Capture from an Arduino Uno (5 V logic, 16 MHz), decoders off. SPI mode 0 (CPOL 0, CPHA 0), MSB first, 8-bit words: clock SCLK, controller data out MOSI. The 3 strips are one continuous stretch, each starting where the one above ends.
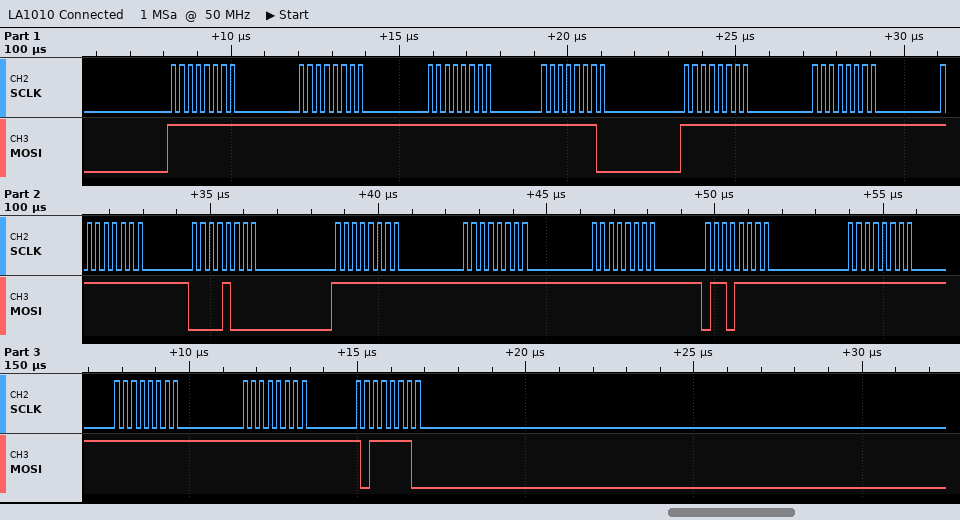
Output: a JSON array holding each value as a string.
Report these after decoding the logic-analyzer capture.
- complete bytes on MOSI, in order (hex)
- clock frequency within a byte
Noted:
["0xFF 0xFF 0xFF 0xFE 0xFF 0xFF 0xFF 0x08 0xFF 0xFF 0xFF 0x6F 0xFF 0xFF 0xFF 0xBE", "4 MHz"]
